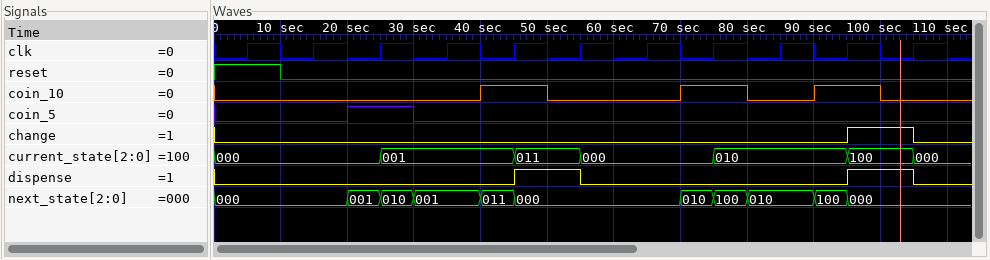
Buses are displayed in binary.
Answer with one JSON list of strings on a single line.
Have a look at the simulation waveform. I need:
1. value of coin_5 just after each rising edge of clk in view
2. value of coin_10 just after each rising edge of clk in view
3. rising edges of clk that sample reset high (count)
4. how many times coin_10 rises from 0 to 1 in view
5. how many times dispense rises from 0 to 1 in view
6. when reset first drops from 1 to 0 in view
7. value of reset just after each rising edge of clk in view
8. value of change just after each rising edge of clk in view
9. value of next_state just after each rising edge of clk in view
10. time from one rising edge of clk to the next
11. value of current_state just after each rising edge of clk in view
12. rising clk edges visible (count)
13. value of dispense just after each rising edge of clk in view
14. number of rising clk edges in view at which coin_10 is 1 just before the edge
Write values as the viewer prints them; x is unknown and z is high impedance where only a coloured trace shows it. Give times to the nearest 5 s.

["0 0 1 0 0 0 0 0 0 0 0", "0 0 0 0 1 0 0 1 0 1 0", "1", "3", "2", "10 s", "1 0 0 0 0 0 0 0 0 0 0", "0 0 0 0 0 0 0 0 0 1 0", "000, 000, 010, 001, 000, 000, 000, 100, 010, 000, 000", "10 s", "000, 000, 001, 001, 011, 000, 000, 010, 010, 100, 000", "11", "0 0 0 0 1 0 0 0 0 1 0", "3"]
